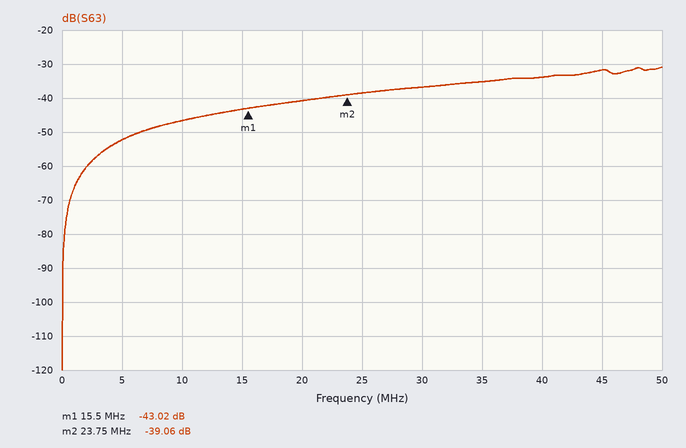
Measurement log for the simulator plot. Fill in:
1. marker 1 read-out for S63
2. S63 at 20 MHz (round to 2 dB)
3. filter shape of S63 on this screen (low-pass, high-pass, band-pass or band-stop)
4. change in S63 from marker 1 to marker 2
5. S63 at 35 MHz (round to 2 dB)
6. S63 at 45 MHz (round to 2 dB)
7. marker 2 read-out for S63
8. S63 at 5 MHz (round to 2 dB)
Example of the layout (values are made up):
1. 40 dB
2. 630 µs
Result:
1. -43.02 dB
2. -40 dB
3. high-pass
4. 3.96 dB
5. -36 dB
6. -32 dB
7. -39.06 dB
8. -52 dB
